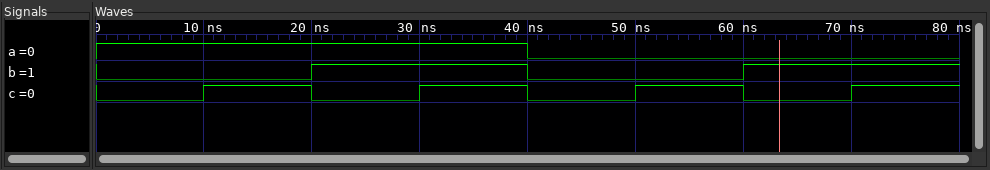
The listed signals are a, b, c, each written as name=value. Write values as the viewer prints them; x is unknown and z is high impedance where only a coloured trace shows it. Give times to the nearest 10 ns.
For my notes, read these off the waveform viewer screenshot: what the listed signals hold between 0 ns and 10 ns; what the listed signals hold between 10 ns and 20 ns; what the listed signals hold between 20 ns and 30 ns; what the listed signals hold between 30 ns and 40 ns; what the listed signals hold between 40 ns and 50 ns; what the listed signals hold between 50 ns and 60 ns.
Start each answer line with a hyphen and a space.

- a=1, b=0, c=0
- a=1, b=0, c=1
- a=1, b=1, c=0
- a=1, b=1, c=1
- a=0, b=0, c=0
- a=0, b=0, c=1
